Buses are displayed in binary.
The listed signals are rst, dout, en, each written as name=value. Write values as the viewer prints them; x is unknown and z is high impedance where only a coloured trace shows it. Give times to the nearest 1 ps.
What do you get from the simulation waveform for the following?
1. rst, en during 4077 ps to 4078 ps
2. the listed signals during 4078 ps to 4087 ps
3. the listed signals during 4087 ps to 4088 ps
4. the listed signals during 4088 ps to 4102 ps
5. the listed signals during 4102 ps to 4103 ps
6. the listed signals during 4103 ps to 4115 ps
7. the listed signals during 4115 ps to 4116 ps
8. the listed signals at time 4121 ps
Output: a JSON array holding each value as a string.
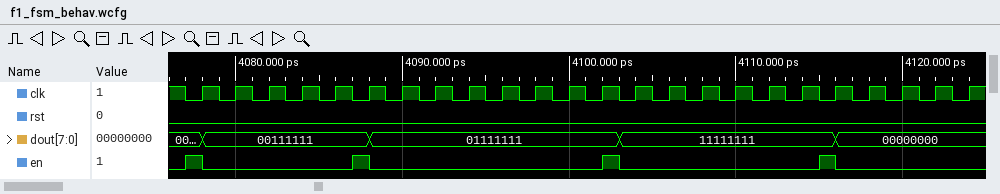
["rst=0, en=1", "rst=0, dout=00111111, en=0", "rst=0, dout=00111111, en=1", "rst=0, dout=01111111, en=0", "rst=0, dout=01111111, en=1", "rst=0, dout=11111111, en=0", "rst=0, dout=11111111, en=1", "rst=0, dout=00000000, en=0"]
